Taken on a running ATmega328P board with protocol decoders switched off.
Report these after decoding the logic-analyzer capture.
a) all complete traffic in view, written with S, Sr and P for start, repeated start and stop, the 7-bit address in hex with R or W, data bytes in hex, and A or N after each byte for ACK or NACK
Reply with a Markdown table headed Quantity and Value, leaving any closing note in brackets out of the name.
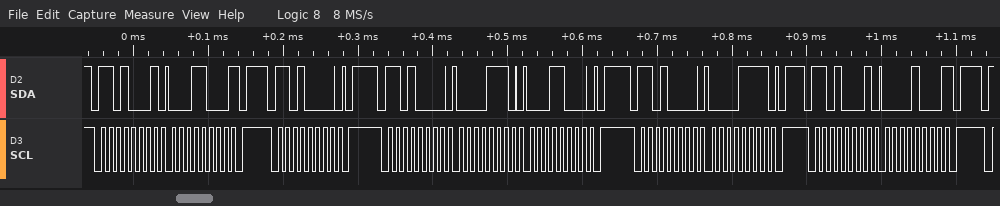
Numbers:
| Quantity | Value |
|---|---|
| all complete traffic in view, written with S, Sr and P for start, repeated start and stop, the 7-bit address in hex with R or W, data bytes in hex, and A or N after each byte for ACK or NACK | S 68R A 18 N P S 68W A P S 68W A 0E A 18 A P S 68W A 0F A P S 68R A 08 N P |
